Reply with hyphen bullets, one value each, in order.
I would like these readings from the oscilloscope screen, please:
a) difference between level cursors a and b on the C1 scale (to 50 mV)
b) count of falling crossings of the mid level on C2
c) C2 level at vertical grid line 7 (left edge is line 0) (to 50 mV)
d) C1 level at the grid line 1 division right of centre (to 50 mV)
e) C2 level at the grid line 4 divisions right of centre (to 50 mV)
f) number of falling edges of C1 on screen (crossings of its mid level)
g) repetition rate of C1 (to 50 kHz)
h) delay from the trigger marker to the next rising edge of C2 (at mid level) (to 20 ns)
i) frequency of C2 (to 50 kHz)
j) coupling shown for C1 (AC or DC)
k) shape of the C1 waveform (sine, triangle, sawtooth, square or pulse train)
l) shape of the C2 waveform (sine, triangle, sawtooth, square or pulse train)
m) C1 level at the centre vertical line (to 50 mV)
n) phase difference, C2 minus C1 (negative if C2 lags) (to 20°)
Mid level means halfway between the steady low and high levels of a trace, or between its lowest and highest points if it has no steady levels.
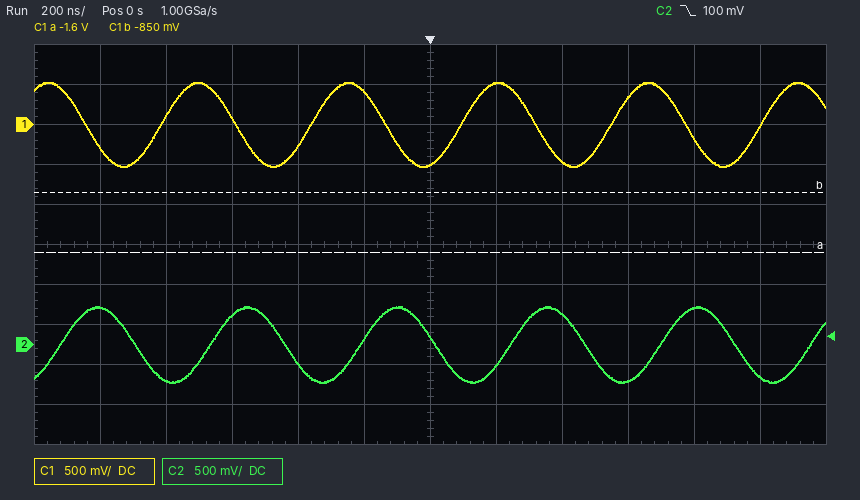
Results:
- 750 mV
- 5
- -250 mV
- 500 mV
- 450 mV
- 5
- 2.20 MHz
- 240 ns
- 2.20 MHz
- DC
- sine
- sine
- -500 mV
- -120°
